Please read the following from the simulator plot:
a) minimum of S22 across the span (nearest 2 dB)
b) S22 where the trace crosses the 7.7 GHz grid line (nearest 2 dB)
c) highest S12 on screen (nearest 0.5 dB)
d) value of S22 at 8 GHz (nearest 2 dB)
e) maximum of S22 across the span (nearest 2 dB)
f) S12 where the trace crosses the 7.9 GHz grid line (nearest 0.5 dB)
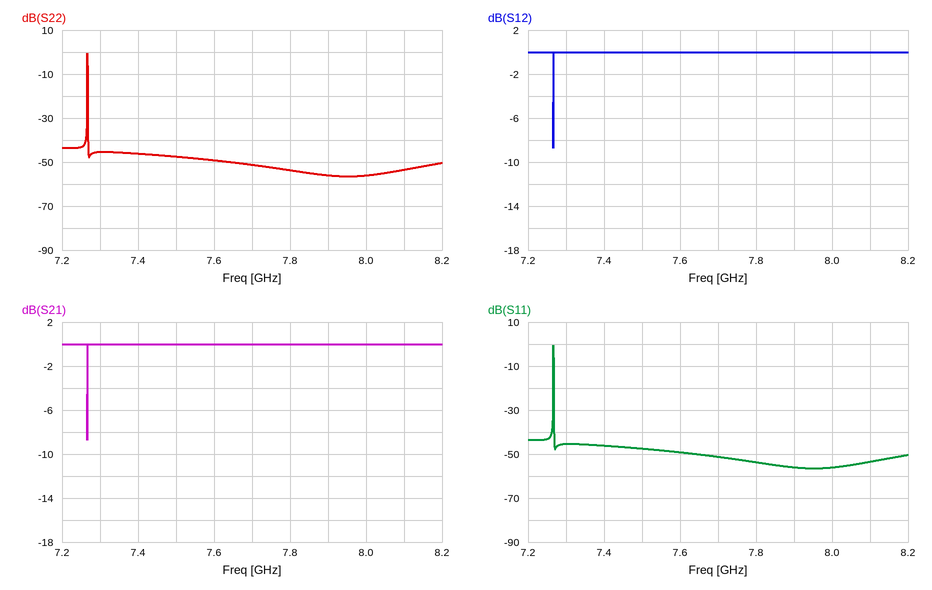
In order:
-56 dB
-52 dB
0.0 dB
-56 dB
0 dB
0.0 dB
